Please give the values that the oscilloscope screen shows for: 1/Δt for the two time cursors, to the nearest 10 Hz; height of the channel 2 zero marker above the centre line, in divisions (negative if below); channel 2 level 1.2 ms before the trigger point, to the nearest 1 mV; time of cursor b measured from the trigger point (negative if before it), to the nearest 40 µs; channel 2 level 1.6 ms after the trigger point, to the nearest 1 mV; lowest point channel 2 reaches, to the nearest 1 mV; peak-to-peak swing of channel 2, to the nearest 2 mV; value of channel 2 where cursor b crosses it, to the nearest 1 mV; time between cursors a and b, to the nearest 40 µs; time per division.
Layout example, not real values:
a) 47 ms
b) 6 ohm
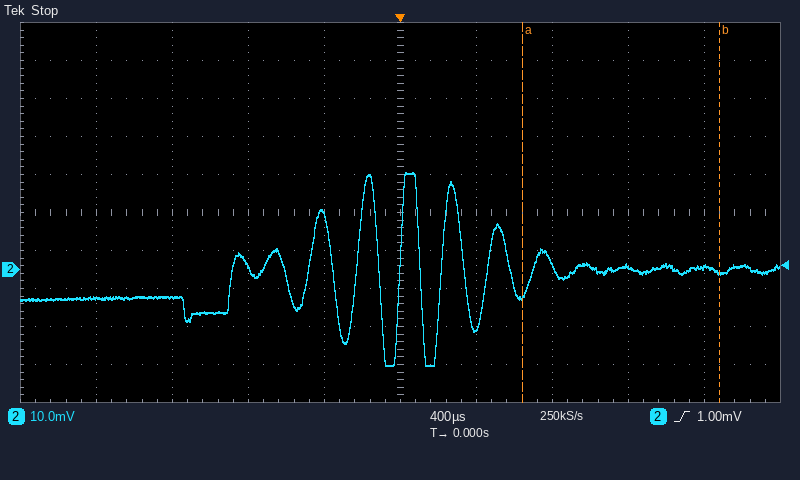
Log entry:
a) 960 Hz
b) -1.5 div
c) -7 mV
d) +1.68 ms
e) 1 mV
f) -25 mV
g) 50 mV
h) -1 mV
i) 1.04 ms
j) 400 µs
